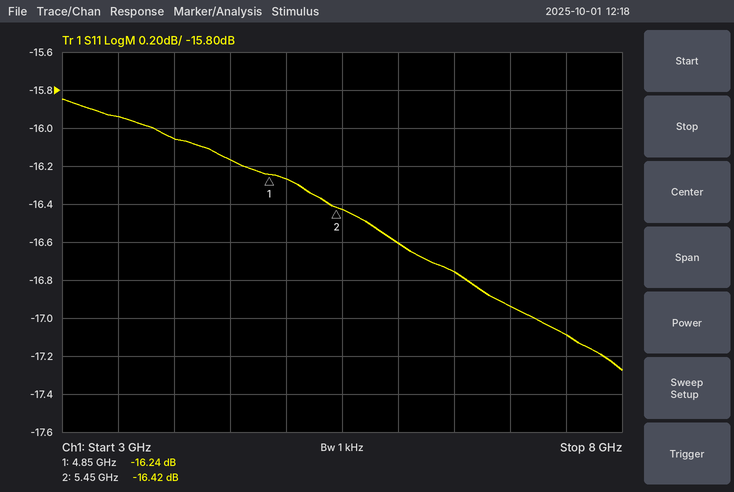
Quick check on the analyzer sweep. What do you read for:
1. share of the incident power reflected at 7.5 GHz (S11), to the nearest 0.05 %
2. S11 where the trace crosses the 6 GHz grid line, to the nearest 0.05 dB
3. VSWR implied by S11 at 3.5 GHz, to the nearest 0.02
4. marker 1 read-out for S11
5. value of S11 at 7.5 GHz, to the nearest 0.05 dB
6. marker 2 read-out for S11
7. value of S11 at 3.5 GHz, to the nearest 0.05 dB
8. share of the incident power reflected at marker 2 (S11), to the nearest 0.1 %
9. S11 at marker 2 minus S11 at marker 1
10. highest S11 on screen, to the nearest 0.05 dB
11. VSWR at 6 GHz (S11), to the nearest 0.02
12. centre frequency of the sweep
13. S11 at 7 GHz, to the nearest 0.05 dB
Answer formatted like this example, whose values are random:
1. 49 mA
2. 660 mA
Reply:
1. 1.95 %
2. -16.60 dB
3. 1.38
4. -16.24 dB
5. -17.10 dB
6. -16.42 dB
7. -15.95 dB
8. 2.3 %
9. -0.18 dB
10. -15.85 dB
11. 1.34
12. 5.5 GHz
13. -16.95 dB
